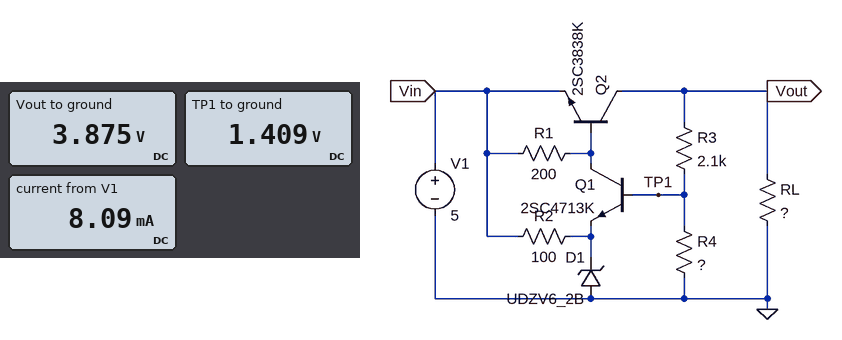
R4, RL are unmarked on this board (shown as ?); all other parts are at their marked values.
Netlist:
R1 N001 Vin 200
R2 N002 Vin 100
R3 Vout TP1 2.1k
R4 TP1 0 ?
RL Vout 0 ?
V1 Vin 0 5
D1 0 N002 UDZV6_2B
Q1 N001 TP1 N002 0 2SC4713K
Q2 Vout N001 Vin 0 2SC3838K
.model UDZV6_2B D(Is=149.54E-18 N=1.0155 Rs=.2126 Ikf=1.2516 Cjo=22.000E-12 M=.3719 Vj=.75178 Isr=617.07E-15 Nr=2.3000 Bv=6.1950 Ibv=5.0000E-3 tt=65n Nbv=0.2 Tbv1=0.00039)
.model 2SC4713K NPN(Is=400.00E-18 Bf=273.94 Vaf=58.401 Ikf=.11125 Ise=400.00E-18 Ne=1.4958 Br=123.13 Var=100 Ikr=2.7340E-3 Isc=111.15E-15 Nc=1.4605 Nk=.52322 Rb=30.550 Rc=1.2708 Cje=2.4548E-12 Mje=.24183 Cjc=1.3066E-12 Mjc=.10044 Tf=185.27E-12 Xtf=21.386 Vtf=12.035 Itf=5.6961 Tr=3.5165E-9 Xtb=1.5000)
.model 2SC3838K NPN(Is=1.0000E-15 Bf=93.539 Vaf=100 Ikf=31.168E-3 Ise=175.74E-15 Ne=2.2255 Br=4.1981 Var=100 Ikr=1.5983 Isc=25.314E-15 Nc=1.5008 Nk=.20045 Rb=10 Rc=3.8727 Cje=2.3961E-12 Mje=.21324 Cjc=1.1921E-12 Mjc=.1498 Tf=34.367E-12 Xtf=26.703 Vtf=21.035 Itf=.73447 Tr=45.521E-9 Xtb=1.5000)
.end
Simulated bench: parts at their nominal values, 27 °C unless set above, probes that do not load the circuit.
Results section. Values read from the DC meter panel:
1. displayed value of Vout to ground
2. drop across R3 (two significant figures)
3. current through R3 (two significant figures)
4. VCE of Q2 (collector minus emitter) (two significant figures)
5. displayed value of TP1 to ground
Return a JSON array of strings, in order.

["3.875 V", "2.5 V", "1.2 mA", "-1.1 V", "1.409 V"]
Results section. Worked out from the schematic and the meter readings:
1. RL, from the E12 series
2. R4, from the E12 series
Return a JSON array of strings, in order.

["560 Ω", "1.2 kΩ"]
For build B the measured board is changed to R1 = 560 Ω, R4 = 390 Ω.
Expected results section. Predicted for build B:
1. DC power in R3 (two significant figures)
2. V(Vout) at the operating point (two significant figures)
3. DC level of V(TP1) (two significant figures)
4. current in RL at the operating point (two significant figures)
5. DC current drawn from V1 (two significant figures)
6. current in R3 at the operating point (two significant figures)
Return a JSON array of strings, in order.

["3.9 mW", "3.4 V", "530 mV", "6.1 mA", "7.4 mA", "1.4 mA"]
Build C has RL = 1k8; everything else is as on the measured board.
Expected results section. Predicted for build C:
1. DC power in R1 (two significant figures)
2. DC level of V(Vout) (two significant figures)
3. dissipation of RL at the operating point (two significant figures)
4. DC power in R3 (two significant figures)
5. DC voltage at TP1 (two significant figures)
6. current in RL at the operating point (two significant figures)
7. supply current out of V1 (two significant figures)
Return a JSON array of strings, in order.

["94 µW", "4.1 V", "9.3 mW", "3.2 mW", "1.5 V", "2.3 mA", "3.5 mA"]
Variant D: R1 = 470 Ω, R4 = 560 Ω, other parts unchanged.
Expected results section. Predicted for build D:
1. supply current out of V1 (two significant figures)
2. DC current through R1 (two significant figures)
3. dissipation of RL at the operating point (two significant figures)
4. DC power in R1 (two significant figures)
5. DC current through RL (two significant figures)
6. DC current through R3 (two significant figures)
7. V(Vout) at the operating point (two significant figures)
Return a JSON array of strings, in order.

["7.6 mA", "1.5 mA", "22 mW", "1.0 mW", "6.3 mA", "1.3 mA", "3.5 V"]
